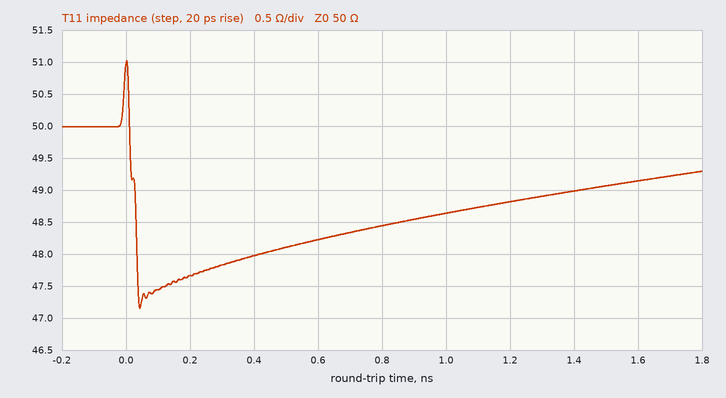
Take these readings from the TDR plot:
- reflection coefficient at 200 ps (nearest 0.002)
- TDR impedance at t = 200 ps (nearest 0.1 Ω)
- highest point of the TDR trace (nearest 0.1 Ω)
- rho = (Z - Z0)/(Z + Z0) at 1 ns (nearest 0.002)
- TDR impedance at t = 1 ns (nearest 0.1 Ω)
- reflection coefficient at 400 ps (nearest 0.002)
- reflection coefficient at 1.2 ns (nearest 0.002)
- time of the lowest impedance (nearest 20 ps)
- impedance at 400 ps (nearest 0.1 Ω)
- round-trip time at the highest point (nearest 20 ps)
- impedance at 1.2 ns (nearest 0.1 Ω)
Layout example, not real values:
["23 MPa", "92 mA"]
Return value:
["-0.024", "47.7 Ω", "51.0 Ω", "-0.014", "48.6 Ω", "-0.020", "-0.012", "40 ps", "48.0 Ω", "0 ps", "48.8 Ω"]
